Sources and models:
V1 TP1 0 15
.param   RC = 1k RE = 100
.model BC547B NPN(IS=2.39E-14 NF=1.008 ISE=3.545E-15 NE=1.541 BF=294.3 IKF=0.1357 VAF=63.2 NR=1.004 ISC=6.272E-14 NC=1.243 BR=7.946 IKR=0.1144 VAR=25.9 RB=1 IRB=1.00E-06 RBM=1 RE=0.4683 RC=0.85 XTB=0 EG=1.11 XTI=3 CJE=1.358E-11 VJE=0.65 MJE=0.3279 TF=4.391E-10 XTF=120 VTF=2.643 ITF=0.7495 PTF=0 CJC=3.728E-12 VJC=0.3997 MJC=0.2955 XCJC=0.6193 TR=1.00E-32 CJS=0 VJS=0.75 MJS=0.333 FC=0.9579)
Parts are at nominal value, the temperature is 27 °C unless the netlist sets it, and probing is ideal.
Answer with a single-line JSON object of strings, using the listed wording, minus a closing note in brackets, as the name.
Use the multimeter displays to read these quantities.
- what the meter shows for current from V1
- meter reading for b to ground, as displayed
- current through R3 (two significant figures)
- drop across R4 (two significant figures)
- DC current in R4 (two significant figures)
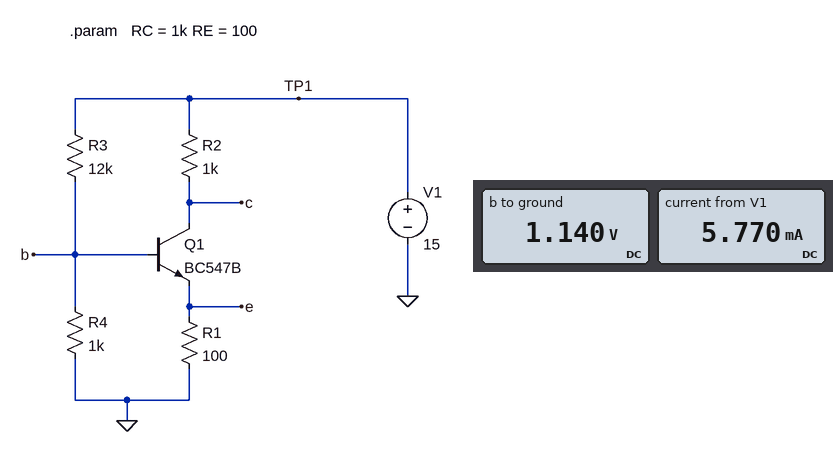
{"what the meter shows for current from V1": "5.770 mA", "meter reading for b to ground, as displayed": "1.140 V", "current through R3": "1.2 mA", "drop across R4": "1.1 V", "DC current in R4": "1.1 mA"}
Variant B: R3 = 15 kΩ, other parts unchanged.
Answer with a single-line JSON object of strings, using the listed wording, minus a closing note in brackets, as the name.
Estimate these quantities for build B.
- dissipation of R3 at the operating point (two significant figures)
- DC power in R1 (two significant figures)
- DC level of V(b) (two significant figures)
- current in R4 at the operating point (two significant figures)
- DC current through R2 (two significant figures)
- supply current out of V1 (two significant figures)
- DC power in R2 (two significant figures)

{"dissipation of R3 at the operating point": "13 mW", "DC power in R1": "720 µW", "DC level of V(b)": "930 mV", "current in R4 at the operating point": "930 µA", "DC current through R2": "2.7 mA", "supply current out of V1": "3.6 mA", "DC power in R2": "7.2 mW"}
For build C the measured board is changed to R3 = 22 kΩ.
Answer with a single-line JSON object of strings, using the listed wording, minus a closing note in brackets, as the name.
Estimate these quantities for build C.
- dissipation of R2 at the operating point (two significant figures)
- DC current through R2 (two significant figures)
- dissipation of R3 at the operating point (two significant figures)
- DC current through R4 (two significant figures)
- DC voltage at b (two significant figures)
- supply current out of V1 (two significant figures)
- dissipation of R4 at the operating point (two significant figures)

{"dissipation of R2 at the operating point": "170 µW", "DC current through R2": "410 µA", "dissipation of R3 at the operating point": "9.4 mW", "DC current through R4": "650 µA", "DC voltage at b": "650 mV", "supply current out of V1": "1.1 mA", "dissipation of R4 at the operating point": "420 µW"}
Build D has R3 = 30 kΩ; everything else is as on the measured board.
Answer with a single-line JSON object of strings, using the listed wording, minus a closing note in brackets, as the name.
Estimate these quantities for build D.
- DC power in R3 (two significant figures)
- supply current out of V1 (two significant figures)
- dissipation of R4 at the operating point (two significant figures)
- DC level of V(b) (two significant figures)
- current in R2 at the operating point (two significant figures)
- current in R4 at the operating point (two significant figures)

{"DC power in R3": "7.0 mW", "supply current out of V1": "490 µA", "dissipation of R4 at the operating point": "230 µW", "DC level of V(b)": "480 mV", "current in R2 at the operating point": "3.3 µA", "current in R4 at the operating point": "480 µA"}
